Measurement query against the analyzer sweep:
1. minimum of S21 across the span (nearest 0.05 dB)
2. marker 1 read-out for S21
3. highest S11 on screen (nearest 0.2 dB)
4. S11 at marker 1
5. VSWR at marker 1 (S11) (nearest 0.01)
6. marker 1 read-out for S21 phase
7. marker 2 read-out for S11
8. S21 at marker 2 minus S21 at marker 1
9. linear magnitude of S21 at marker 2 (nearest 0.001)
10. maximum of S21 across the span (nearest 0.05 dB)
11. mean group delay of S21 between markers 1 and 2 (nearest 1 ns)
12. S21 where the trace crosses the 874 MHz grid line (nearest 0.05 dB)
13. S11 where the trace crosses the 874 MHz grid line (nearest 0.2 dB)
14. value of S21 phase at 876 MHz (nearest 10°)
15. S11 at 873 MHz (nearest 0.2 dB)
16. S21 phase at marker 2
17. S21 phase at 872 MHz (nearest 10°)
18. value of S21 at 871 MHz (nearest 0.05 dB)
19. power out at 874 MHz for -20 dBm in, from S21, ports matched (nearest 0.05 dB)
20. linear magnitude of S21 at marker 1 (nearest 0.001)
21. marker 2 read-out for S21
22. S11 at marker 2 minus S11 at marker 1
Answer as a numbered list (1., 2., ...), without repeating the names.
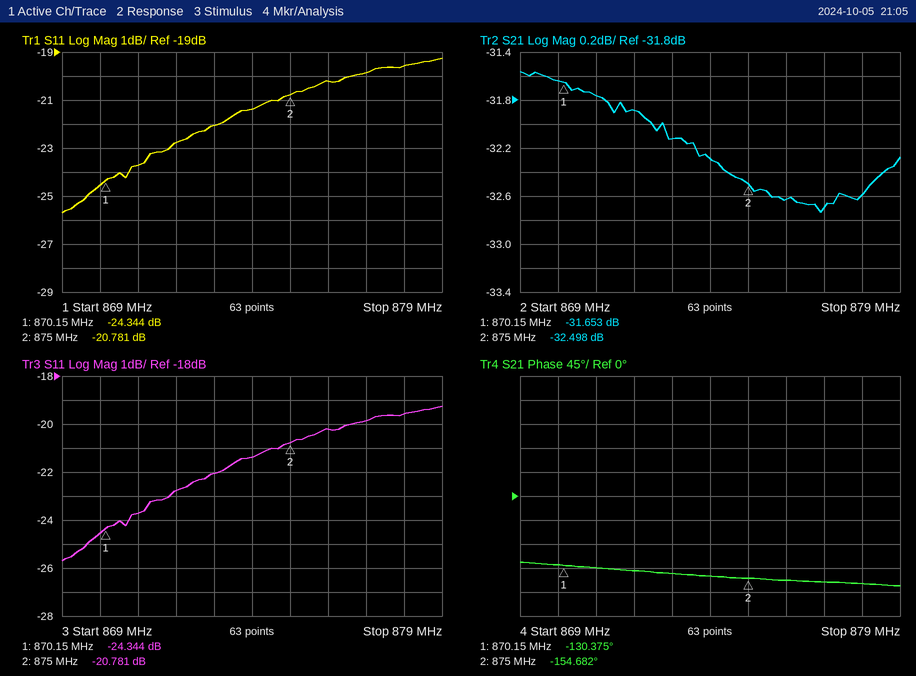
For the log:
1. -32.75 dB
2. -31.653 dB
3. -19.2 dB
4. -24.344 dB
5. 1.13
6. -130.375°
7. -20.781 dB
8. -0.845 dB
9. 0.024
10. -31.55 dB
11. 14 ns
12. -32.30 dB
13. -21.4 dB
14. -160°
15. -22.0 dB
16. -154.682°
17. -140°
18. -31.75 dB
19. -52.30 dBm
20. 0.026
21. -32.498 dB
22. 3.563 dB
